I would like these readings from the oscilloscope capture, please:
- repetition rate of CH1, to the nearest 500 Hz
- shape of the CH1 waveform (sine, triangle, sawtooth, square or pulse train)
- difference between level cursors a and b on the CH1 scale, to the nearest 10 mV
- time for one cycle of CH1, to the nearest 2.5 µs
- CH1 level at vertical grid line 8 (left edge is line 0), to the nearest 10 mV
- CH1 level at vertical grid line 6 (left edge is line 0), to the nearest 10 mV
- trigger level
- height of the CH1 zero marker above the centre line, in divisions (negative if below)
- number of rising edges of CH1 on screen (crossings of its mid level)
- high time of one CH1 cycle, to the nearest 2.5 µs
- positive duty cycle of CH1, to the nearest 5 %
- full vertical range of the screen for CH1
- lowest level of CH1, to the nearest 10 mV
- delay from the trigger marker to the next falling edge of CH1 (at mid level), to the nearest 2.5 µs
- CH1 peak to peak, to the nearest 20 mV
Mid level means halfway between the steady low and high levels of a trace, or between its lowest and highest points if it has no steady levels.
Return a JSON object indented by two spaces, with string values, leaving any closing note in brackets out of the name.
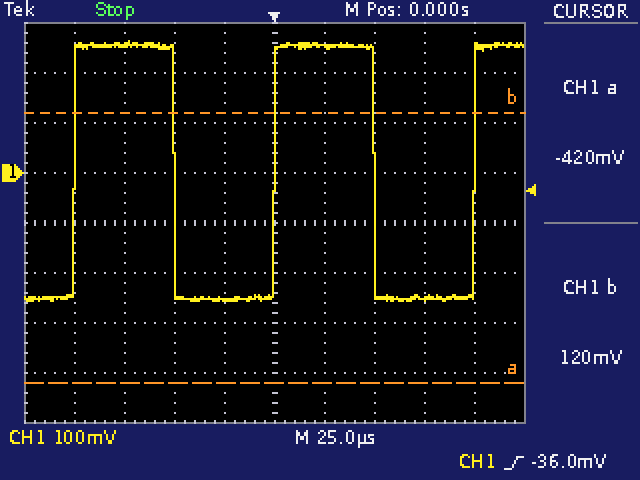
{
  "repetition rate of CH1, to the nearest 500 Hz": "10.0 kHz",
  "shape of the CH1 waveform": "square",
  "difference between level cursors a and b on the CH1 scale, to the nearest 10 mV": "540 mV",
  "time for one cycle of CH1, to the nearest 2.5 µs": "100.0 µs",
  "CH1 level at vertical grid line 8 (left edge is line 0), to the nearest 10 mV": "-250 mV",
  "CH1 level at vertical grid line 6 (left edge is line 0), to the nearest 10 mV": "250 mV",
  "trigger level": "-36.0 mV",
  "height of the CH1 zero marker above the centre line, in divisions": "+1.0 div",
  "number of rising edges of CH1 on screen": "3",
  "high time of one CH1 cycle, to the nearest 2.5 µs": "50.0 µs",
  "positive duty cycle of CH1, to the nearest 5 %": "50 %",
  "full vertical range of the screen for CH1": "800 mV",
  "lowest level of CH1, to the nearest 10 mV": "-260 mV",
  "delay from the trigger marker to the next falling edge of CH1 (at mid level), to the nearest 2.5 µs": "50.0 µs",
  "CH1 peak to peak, to the nearest 20 mV": "520 mV"
}
